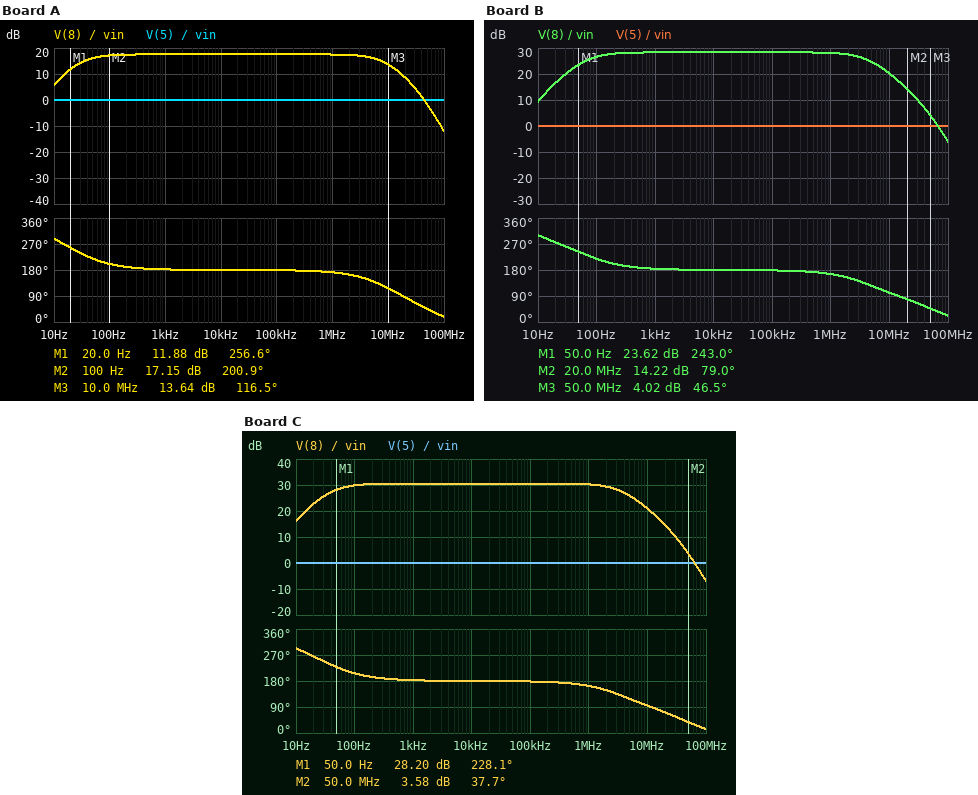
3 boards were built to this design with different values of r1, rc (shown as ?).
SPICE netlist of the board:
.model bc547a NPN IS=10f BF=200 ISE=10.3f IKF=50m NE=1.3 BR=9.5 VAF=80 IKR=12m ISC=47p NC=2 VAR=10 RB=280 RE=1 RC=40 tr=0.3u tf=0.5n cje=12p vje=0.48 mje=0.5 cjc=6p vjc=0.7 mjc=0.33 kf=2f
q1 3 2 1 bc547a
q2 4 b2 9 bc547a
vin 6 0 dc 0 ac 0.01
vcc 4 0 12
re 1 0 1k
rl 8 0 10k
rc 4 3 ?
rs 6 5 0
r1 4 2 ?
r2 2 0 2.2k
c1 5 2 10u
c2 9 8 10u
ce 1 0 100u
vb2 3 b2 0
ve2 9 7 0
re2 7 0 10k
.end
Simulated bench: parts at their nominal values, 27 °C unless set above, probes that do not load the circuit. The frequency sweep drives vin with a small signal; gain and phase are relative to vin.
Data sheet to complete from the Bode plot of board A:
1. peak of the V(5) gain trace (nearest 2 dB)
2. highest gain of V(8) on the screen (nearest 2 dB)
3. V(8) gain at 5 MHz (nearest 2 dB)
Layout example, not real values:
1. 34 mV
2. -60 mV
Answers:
1. 0 dB
2. 18 dB
3. 16 dB
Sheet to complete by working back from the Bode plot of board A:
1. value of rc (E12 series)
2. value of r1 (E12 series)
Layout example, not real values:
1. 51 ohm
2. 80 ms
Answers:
1. 470 Ω
2. 22 kΩ
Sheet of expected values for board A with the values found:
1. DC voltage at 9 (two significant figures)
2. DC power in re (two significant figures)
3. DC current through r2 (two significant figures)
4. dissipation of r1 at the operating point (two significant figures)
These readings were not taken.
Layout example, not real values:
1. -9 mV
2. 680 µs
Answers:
1. 11 V
2. 200 µW
3. 490 µA
4. 5.4 mW
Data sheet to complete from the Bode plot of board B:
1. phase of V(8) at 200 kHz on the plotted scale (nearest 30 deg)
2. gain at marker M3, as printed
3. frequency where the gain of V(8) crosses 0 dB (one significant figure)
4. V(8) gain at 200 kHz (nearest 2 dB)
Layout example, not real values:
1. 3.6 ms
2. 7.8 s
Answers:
1. 180 deg
2. 4.02 dB
3. 70 MHz
4. 28 dB
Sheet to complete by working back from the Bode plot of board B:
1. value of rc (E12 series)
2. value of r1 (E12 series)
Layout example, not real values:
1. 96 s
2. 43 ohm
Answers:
1. 680 Ω
2. 12 kΩ
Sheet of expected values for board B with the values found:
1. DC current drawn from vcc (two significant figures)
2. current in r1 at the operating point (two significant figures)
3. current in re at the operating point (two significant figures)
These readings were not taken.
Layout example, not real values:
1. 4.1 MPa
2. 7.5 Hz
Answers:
1. 3.1 mA
2. 850 µA
3. 1.2 mA
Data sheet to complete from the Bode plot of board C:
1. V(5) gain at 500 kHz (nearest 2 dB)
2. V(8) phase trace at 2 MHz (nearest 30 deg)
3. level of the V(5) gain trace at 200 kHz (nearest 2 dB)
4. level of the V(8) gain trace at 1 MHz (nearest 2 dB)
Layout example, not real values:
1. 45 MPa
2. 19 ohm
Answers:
1. 0 dB
2. 150 deg
3. 0 dB
4. 30 dB
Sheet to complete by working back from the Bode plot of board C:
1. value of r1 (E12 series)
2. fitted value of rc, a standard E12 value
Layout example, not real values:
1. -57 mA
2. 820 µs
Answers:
1. 18 kΩ
2. 1.5 kΩ
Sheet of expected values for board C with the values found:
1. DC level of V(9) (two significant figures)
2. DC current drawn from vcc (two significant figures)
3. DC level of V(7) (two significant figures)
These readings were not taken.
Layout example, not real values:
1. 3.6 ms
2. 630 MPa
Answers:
1. 10 V
2. 2.3 mA
3. 10 V
